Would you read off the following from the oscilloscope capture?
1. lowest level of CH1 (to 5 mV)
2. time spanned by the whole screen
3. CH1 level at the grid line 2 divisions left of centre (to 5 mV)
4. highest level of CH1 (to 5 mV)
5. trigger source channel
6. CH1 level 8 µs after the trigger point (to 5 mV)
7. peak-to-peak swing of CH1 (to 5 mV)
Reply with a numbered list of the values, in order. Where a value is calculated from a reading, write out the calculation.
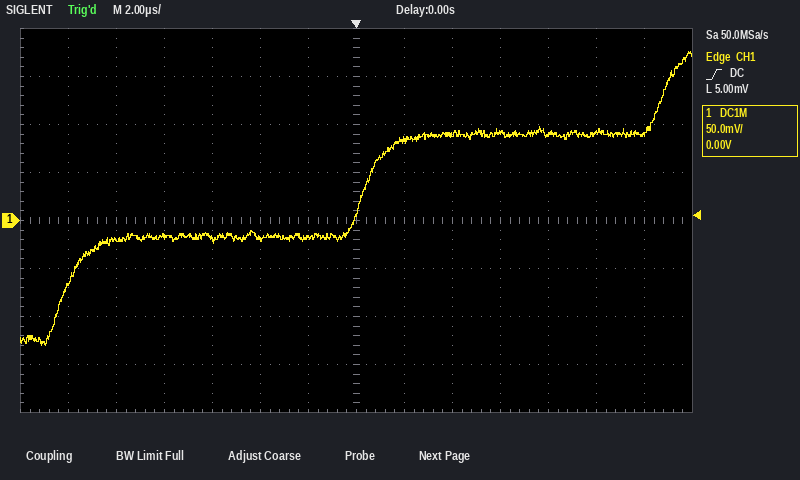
1. -130 mV
2. 28 µs
3. -20 mV
4. 175 mV
5. CH1
6. 90 mV
7. 175 mV − (-130 mV) = 305 mV
